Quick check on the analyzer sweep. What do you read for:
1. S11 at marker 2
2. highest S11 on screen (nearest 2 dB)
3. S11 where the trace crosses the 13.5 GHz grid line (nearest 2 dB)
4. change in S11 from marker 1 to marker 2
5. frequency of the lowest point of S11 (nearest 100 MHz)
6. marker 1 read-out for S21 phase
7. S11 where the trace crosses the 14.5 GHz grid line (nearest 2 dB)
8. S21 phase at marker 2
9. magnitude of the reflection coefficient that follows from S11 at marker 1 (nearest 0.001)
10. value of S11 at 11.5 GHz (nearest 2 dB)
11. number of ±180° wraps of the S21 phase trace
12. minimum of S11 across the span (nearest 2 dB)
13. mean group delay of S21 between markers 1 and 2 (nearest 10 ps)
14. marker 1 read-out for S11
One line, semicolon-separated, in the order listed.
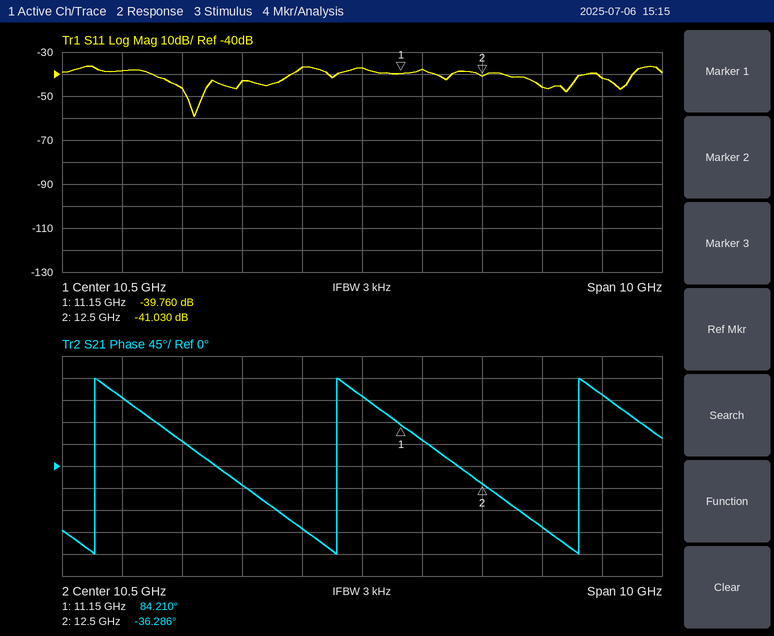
-41.030 dB; -36 dB; -46 dB; -1.270 dB; 7.7 GHz; 84.210°; -42 dB; -36.286°; 0.010; -38 dB; 3; -60 dB; 250 ps; -39.760 dB
